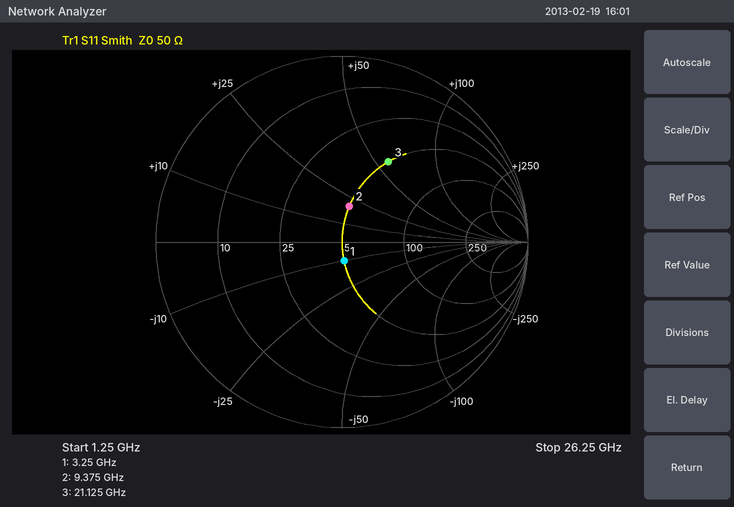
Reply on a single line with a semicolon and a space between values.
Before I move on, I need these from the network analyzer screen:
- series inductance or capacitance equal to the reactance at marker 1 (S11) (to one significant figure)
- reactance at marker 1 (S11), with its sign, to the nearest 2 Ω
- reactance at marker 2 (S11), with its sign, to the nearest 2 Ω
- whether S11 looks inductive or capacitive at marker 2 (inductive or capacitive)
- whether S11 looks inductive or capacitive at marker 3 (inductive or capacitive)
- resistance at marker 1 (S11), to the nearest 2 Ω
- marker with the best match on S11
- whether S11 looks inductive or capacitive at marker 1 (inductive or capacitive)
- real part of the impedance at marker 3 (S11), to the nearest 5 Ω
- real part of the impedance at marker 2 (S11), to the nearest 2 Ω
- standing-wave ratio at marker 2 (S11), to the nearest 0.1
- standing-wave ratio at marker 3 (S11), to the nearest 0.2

5 pF; -10 Ω; +20 Ω; inductive; inductive; 50 Ω; marker 1; capacitive; 50 Ω; 50 Ω; 1.5; 3.0
